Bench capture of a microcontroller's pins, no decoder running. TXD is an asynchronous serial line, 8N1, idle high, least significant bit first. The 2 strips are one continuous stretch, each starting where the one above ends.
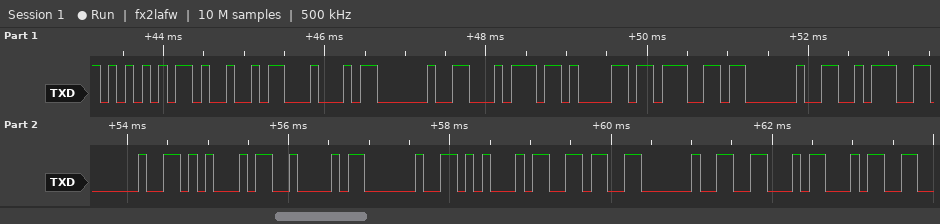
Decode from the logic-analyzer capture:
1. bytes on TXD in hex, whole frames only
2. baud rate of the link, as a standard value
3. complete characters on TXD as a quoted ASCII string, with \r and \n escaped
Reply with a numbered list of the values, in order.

1. 55 49 44 20 74 61 67 20 3A 20 45 42 20 45 36 20 46 34
2. 9600 baud
3. "UID tag : EB E6 F4"
